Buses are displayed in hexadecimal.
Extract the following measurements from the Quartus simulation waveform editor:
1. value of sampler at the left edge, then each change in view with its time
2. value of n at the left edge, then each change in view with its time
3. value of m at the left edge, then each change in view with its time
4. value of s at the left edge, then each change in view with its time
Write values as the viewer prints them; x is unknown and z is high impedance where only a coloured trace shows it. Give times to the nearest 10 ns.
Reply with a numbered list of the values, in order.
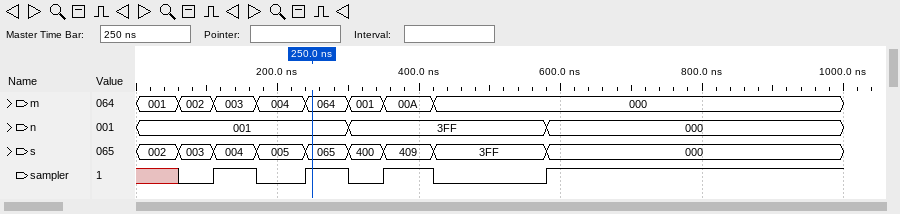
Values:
1. x, 0 at 60 ns, 1 at 110 ns, 0 at 170 ns, 1 at 240 ns, 0 at 300 ns, 1 at 350 ns, 0 at 420 ns, 1 at 580 ns
2. 001, 3FF at 300 ns, 000 at 580 ns
3. 001, 002 at 60 ns, 003 at 110 ns, 004 at 170 ns, 064 at 240 ns, 001 at 300 ns, 00A at 350 ns, 000 at 420 ns
4. 002, 003 at 60 ns, 004 at 110 ns, 005 at 170 ns, 065 at 240 ns, 400 at 300 ns, 409 at 350 ns, 3FF at 420 ns, 000 at 580 ns
